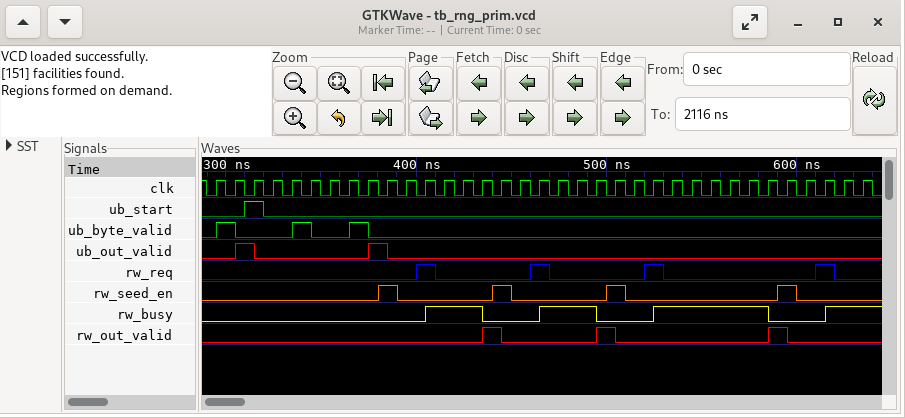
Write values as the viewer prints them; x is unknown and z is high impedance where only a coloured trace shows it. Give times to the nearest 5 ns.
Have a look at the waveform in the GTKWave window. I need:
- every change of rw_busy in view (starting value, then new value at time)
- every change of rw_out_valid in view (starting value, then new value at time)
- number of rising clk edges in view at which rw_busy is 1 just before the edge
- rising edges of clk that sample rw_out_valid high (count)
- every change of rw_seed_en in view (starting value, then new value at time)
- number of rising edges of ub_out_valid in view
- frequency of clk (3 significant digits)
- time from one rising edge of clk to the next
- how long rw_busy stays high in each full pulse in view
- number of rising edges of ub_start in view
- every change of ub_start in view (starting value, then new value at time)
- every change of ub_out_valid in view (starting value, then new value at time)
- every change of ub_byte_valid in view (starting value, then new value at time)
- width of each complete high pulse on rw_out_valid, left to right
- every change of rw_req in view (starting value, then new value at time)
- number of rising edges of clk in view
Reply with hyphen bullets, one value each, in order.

- 0, 1 at 405 ns, 0 at 435 ns, 1 at 465 ns, 0 at 495 ns, 1 at 525 ns, 0 at 585 ns, 1 at 615 ns
- 0, 1 at 435 ns, 0 at 445 ns, 1 at 495 ns, 0 at 505 ns, 1 at 585 ns, 0 at 595 ns
- 14
- 3
- 0, 1 at 380 ns, 0 at 390 ns, 1 at 440 ns, 0 at 450 ns, 1 at 500 ns, 0 at 510 ns, 1 at 590 ns, 0 at 600 ns
- 2
- 100 MHz
- 10 ns
- 30 ns, 30 ns, 60 ns
- 1
- 0, 1 at 310 ns, 0 at 320 ns
- 0, 1 at 305 ns, 0 at 315 ns, 1 at 375 ns, 0 at 385 ns
- 0, 1 at 295 ns, 0 at 305 ns, 1 at 335 ns, 0 at 345 ns, 1 at 365 ns, 0 at 375 ns
- 10 ns, 10 ns, 10 ns
- 0, 1 at 400 ns, 0 at 410 ns, 1 at 460 ns, 0 at 470 ns, 1 at 520 ns, 0 at 530 ns, 1 at 610 ns, 0 at 620 ns
- 35
